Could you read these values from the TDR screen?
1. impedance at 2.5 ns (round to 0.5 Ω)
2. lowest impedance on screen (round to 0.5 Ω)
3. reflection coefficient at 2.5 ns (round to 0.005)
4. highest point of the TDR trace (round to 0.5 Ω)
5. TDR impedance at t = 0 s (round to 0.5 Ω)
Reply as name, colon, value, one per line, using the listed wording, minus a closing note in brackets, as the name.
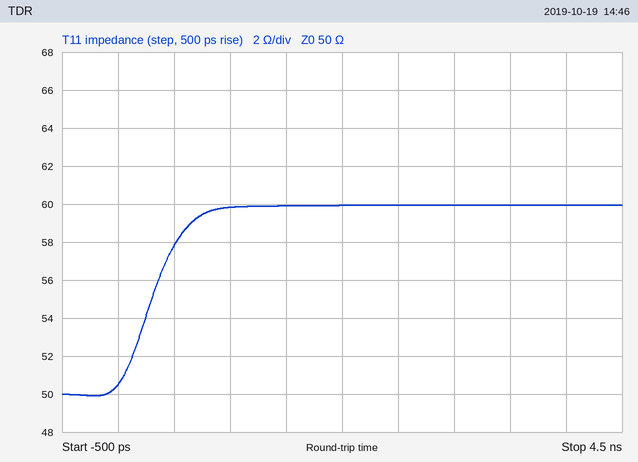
impedance at 2.5 ns: 60.0 Ω
lowest impedance on screen: 50.0 Ω
reflection coefficient at 2.5 ns: +0.090
highest point of the TDR trace: 60.0 Ω
TDR impedance at t = 0 s: 50.5 Ω
